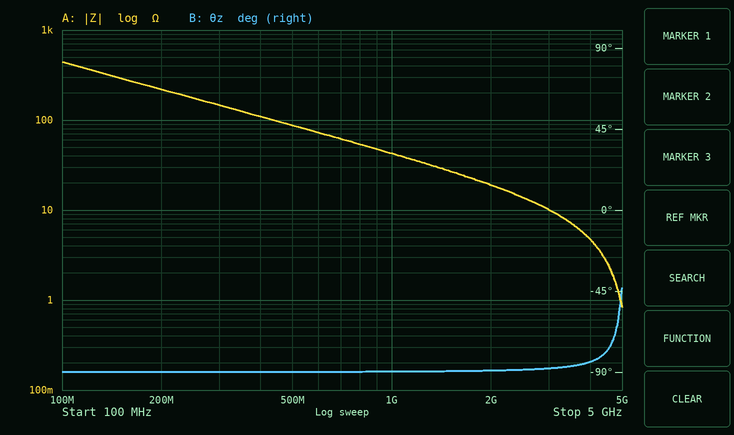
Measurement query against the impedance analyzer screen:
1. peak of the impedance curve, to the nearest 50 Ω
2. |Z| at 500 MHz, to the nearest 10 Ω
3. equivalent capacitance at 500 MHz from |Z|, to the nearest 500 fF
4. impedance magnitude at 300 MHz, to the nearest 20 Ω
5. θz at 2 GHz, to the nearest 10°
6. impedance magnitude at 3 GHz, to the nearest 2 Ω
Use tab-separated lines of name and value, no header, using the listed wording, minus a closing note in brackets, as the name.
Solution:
peak of the impedance curve, to the nearest 50 Ω	450 Ω
|Z| at 500 MHz, to the nearest 10 Ω	90 Ω
equivalent capacitance at 500 MHz from |Z|, to the nearest 500 fF	3.5 pF
impedance magnitude at 300 MHz, to the nearest 20 Ω	140 Ω
θz at 2 GHz, to the nearest 10°	-90°
impedance magnitude at 3 GHz, to the nearest 2 Ω	10 Ω
